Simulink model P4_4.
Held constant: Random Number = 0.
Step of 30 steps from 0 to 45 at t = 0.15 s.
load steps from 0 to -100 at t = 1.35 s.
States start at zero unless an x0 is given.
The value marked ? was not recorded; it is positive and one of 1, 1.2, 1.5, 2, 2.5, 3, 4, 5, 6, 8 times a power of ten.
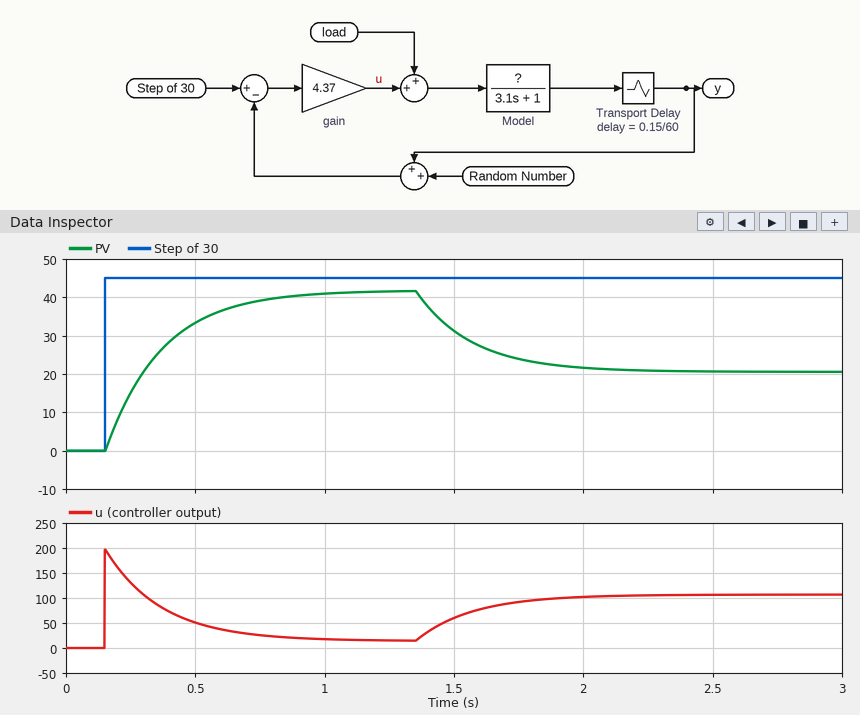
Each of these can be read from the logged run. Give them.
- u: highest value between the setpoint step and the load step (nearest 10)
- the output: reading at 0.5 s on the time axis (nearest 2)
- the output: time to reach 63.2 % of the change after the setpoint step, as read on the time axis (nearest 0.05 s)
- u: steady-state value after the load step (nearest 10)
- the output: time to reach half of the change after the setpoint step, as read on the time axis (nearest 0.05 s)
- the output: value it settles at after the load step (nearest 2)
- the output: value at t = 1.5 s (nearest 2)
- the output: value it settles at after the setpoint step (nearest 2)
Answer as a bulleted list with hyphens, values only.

- 200
- 34
- 0.35 s
- 110
- 0.30 s
- 20
- 32
- 42
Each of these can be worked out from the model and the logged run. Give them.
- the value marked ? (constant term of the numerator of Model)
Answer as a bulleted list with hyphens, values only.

- 3
